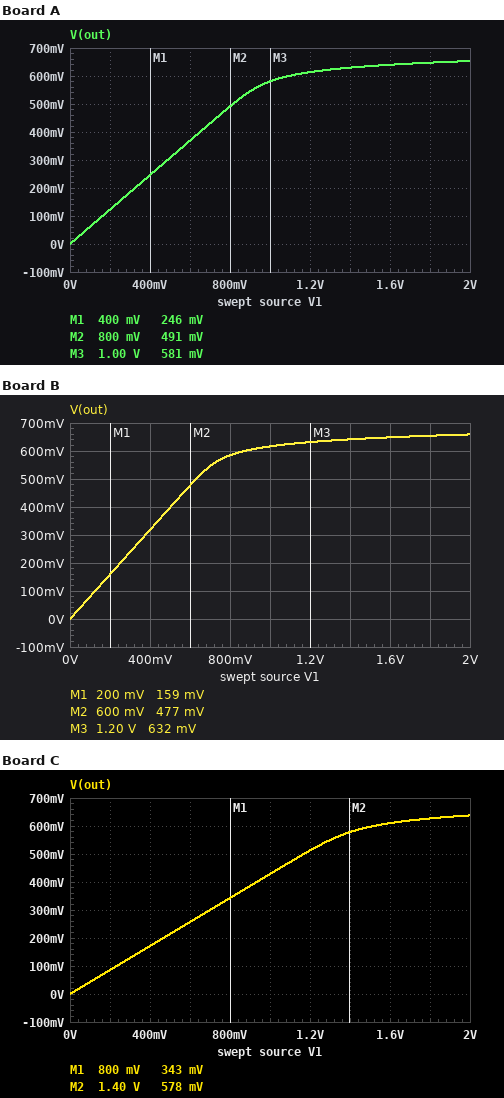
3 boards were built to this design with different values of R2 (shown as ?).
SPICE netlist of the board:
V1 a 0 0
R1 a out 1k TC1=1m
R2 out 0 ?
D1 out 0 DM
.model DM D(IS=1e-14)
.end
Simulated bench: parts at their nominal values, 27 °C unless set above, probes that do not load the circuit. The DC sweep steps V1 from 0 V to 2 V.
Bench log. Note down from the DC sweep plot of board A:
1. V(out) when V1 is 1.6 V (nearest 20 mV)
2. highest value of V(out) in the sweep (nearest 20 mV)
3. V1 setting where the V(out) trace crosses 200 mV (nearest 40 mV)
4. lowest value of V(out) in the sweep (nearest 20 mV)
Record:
640 mV
660 mV
320 mV
0 V
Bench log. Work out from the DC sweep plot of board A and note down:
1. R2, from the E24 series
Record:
1.6 kΩ
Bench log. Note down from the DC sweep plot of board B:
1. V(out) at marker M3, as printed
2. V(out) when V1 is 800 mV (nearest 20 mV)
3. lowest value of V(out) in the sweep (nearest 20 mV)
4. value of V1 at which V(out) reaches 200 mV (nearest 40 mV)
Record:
632 mV
580 mV
0 V
240 mV
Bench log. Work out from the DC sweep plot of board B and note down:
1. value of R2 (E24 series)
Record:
3.9 kΩ
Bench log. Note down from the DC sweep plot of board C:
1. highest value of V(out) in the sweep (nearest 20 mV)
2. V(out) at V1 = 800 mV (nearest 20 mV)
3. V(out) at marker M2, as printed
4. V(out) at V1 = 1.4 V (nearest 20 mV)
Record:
640 mV
340 mV
578 mV
580 mV
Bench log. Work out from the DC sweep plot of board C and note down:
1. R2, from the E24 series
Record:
750 Ω
